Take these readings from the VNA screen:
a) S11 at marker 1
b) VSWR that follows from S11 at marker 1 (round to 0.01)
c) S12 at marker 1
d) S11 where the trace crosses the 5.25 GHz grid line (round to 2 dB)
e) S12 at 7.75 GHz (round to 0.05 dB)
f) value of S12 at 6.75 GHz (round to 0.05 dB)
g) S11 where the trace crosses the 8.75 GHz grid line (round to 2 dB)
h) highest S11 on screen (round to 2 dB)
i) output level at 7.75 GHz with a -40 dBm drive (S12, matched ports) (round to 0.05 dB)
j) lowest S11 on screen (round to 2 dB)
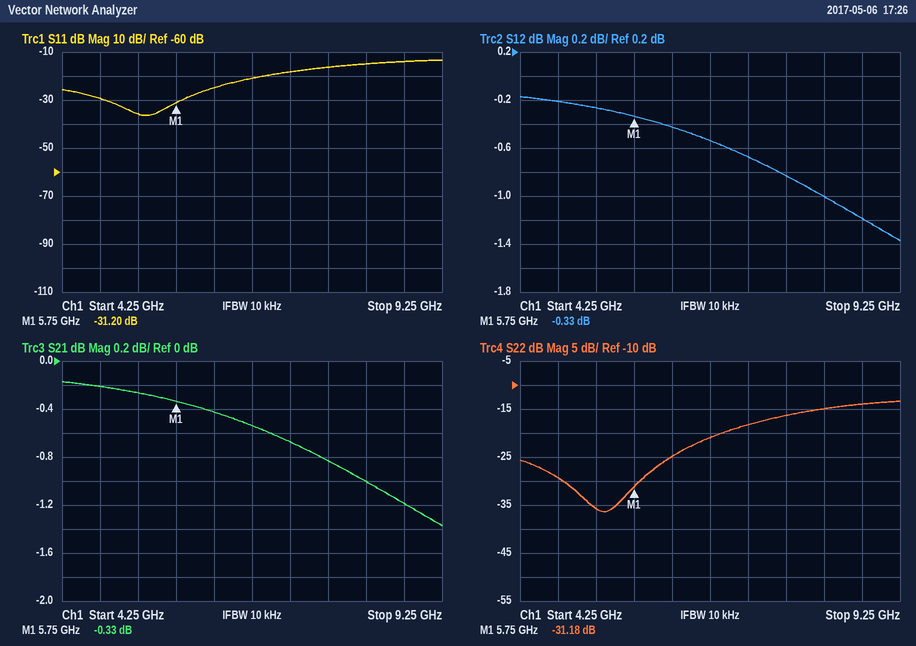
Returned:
-31.20 dB
1.06
-0.33 dB
-36 dB
-0.85 dB
-0.55 dB
-14 dB
-14 dB
-40.85 dBm
-36 dB
